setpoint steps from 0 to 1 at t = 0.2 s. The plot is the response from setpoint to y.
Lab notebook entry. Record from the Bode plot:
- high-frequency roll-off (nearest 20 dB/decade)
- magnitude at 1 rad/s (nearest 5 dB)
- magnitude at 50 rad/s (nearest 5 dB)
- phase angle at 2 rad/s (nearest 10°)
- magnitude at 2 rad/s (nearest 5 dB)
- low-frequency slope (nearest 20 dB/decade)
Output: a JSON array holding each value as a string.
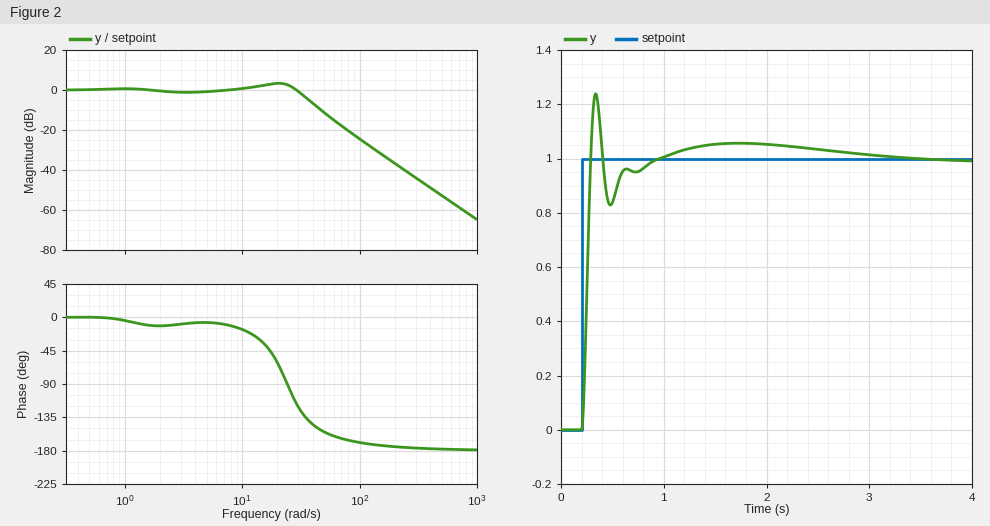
["-40 dB/decade", "0 dB", "-10 dB", "-10°", "0 dB", "0 dB/decade"]
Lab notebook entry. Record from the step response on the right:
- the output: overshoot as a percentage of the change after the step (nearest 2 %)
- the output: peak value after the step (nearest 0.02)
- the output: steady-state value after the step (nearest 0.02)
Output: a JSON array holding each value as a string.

["24 %", "1.24", "1.00"]
